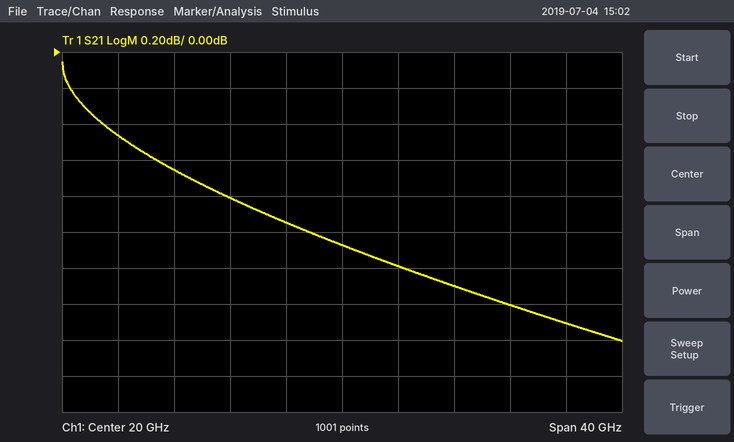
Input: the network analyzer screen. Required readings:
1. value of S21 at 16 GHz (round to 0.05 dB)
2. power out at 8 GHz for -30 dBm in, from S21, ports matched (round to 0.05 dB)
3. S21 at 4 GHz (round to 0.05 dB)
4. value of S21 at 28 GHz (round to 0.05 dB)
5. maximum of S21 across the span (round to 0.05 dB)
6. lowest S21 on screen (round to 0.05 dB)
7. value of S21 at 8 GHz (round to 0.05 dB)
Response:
-0.95 dB
-30.65 dBm
-0.45 dB
-1.30 dB
-0.05 dB
-1.60 dB
-0.65 dB
